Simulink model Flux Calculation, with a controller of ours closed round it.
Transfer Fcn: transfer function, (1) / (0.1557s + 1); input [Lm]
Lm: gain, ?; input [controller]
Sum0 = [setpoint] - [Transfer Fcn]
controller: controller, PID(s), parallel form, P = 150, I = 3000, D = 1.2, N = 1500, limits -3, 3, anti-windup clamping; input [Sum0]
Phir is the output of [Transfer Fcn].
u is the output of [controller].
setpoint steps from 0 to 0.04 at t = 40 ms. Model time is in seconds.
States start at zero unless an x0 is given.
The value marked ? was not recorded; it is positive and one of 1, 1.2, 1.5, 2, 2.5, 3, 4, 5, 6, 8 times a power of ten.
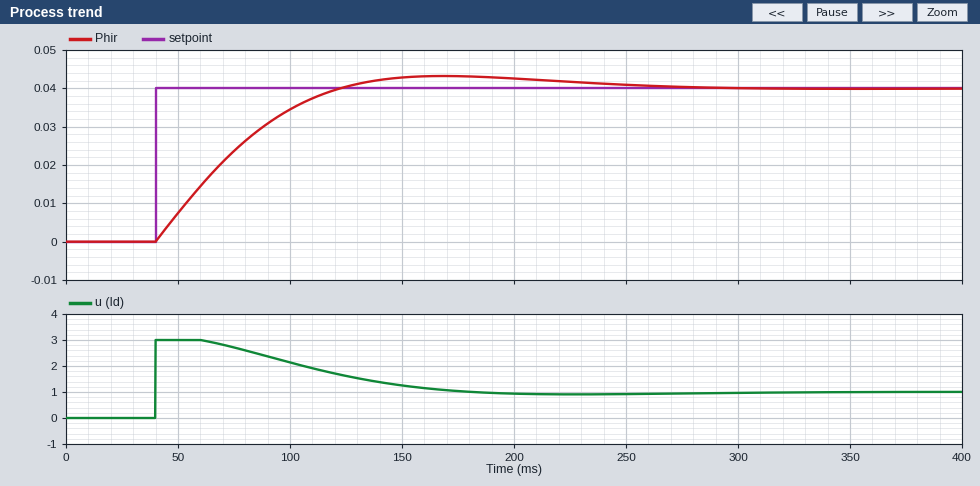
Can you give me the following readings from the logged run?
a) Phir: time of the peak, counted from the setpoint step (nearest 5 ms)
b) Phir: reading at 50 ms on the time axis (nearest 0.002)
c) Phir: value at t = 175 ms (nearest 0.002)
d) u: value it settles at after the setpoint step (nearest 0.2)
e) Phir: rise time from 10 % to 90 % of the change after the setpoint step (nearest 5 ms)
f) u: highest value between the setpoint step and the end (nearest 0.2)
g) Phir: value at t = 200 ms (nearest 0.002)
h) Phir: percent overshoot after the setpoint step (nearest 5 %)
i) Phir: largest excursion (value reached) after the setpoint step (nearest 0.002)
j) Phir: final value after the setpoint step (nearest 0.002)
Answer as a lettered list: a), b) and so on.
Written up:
a) 130 ms
b) 0.008
c) 0.044
d) 1.0
e) 60 ms
f) 3.0
g) 0.042
h) 10 %
i) 0.044
j) 0.040
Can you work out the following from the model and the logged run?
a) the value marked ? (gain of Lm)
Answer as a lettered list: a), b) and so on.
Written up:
a) 0.04
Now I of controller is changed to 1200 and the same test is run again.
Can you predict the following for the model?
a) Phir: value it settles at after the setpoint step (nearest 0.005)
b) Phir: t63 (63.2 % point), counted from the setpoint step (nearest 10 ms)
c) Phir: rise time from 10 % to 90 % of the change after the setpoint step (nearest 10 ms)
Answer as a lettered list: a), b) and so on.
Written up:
a) 0.040
b) 40 ms
c) 80 ms
